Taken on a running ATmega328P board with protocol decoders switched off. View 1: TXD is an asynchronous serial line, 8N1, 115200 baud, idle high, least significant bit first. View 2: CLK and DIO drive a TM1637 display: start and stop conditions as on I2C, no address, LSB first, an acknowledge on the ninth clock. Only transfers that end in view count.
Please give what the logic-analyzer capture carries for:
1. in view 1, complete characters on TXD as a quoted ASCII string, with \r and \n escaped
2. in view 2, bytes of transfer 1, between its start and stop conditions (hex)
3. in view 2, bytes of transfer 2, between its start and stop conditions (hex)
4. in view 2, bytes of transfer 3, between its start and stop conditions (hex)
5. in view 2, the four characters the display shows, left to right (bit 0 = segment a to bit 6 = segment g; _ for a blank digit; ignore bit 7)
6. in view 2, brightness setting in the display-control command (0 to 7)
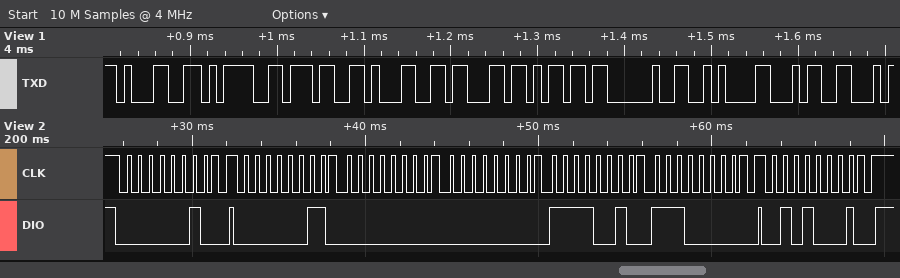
"1=71cm \n4"
40
C0 00 00 4F 07
8A
__37
2
